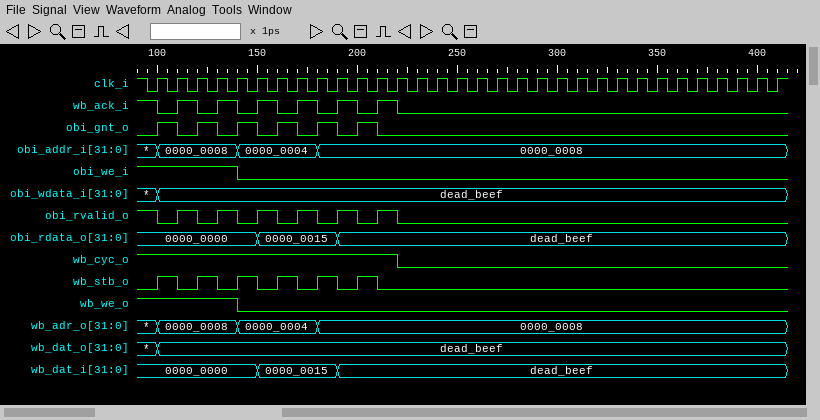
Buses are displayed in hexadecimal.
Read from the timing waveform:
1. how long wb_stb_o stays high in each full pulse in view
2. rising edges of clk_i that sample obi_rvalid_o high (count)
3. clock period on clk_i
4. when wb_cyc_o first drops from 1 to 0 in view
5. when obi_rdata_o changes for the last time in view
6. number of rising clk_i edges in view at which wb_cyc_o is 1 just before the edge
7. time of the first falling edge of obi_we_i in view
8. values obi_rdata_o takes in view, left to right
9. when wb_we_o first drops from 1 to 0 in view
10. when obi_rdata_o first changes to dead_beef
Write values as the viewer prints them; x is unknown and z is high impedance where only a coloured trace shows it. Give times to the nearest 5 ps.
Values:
10 ps, 10 ps, 10 ps, 10 ps, 10 ps, 10 ps
7
10 ps
220 ps
190 ps
13
140 ps
0000_0000, 0000_0015, dead_beef
140 ps
190 ps
